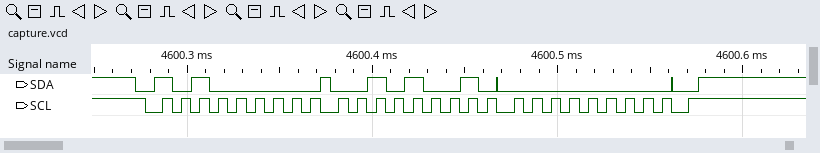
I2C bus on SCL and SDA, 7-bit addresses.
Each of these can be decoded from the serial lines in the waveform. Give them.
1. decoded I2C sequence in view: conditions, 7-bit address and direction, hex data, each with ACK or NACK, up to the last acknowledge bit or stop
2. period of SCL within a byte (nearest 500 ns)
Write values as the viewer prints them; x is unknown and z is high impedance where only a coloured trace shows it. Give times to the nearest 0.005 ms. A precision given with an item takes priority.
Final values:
start, address 50 write ACK, 29 ACK, 00 ACK, stop
10000 ns
